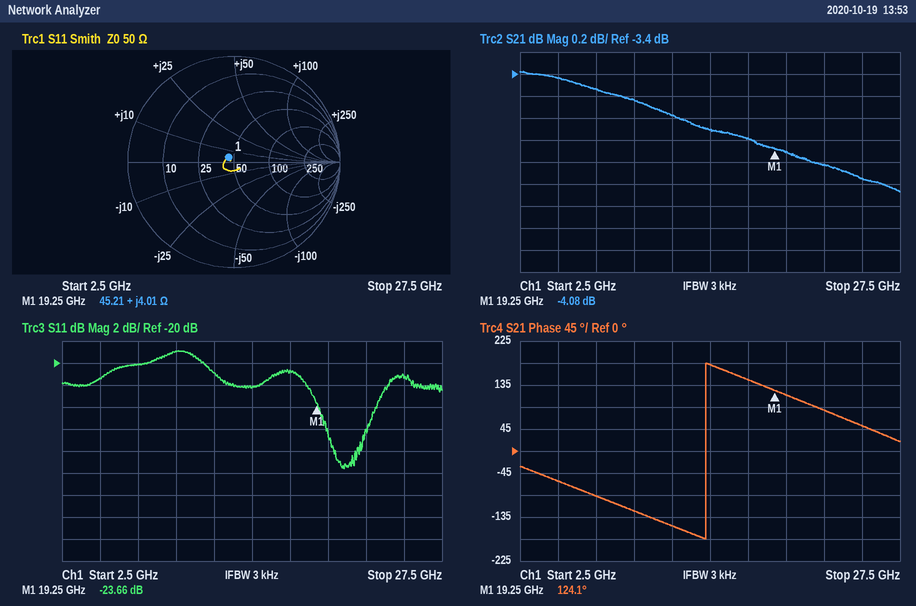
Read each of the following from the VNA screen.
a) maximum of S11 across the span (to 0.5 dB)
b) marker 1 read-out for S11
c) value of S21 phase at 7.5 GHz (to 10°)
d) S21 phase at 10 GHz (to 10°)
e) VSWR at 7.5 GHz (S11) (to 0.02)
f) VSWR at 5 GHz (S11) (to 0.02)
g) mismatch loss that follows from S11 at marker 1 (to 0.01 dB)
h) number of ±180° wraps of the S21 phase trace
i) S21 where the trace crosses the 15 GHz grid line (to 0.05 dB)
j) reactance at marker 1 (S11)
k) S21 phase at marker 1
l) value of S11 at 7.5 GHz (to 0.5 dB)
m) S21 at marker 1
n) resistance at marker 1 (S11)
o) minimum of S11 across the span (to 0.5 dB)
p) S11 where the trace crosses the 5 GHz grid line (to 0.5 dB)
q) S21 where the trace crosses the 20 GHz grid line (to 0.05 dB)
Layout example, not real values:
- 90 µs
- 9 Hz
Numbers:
- -19.0 dB
- -23.66 dB
- -90°
- -120°
- 1.22
- 1.18
- 0.02 dB
- 1
- -3.90 dB
- +4.01 Ω
- 124.1°
- -20.0 dB
- -4.08 dB
- 45.21 Ω
- -29.5 dB
- -21.5 dB
- -4.10 dB
